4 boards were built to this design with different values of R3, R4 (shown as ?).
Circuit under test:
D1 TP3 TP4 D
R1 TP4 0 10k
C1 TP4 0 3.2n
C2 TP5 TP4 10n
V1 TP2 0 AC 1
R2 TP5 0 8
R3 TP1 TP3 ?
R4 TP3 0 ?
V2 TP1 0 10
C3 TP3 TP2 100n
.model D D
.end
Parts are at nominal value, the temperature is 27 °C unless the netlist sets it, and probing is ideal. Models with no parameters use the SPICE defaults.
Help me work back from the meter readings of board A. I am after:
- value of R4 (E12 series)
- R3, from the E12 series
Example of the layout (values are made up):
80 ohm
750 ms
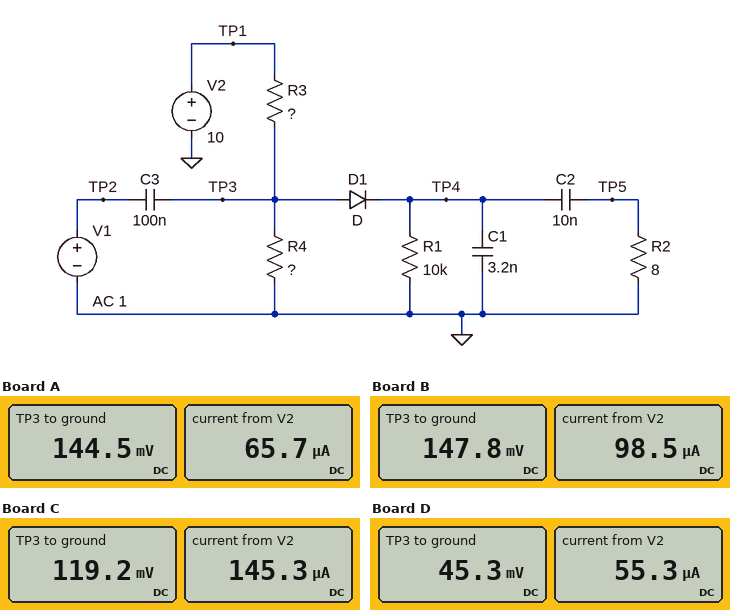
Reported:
2.2 kΩ
150 kΩ
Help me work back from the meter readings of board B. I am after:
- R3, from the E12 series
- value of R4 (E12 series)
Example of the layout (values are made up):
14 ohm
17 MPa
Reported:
100 kΩ
1.5 kΩ
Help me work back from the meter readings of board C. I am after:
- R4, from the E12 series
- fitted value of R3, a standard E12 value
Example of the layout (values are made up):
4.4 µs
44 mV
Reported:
820 Ω
68 kΩ
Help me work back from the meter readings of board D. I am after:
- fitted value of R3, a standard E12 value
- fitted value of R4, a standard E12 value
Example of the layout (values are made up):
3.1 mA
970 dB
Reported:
180 kΩ
820 Ω
